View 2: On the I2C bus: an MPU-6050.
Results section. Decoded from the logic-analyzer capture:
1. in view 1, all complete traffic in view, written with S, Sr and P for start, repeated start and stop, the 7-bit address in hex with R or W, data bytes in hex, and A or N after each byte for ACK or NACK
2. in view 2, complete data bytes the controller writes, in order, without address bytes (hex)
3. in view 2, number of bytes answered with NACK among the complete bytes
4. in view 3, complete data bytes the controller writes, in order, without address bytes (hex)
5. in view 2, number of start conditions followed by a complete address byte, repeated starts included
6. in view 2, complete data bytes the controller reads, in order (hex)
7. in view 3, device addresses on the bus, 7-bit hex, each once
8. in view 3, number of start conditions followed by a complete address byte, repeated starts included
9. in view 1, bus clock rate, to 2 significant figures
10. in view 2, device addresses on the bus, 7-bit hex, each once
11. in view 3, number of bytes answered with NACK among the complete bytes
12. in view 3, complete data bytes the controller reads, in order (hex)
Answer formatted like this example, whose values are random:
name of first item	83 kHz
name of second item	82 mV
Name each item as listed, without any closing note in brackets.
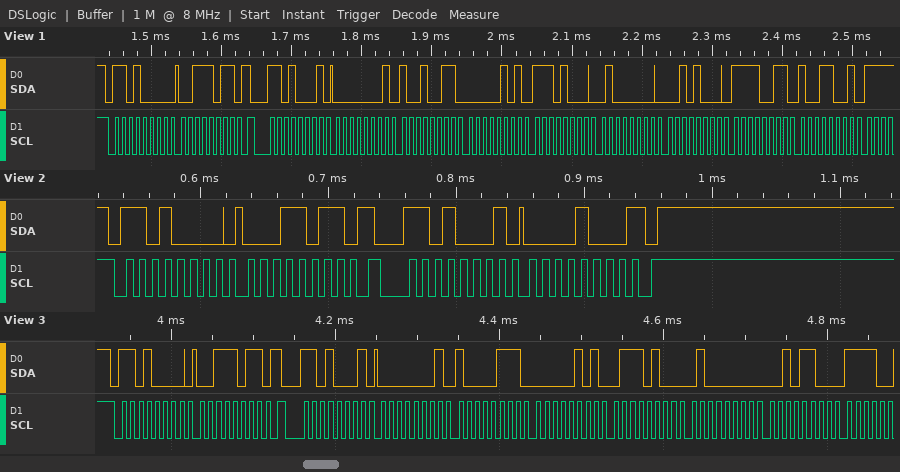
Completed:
in view 1, all complete traffic in view, written with S, Sr and P for start, repeated start and stop, the 7-bit address in hex with R or W, data bytes in hex, and A or N after each byte for ACK or NACK	S 68W A 3B A Sr 68R A 01 A 93 A 05 A E8 A 40 A 28 A F3 A 99 A
in view 2, complete data bytes the controller writes, in order, without address bytes	1B
in view 2, number of bytes answered with NACK among the complete bytes	1
in view 3, complete data bytes the controller writes, in order, without address bytes	3B
in view 2, number of start conditions followed by a complete address byte, repeated starts included	2
in view 2, complete data bytes the controller reads, in order	08
in view 3, device addresses on the bus, 7-bit hex, each once	0x68
in view 3, number of start conditions followed by a complete address byte, repeated starts included	2
in view 1, bus clock rate, to 2 significant figures	100 kHz
in view 2, device addresses on the bus, 7-bit hex, each once	0x68
in view 3, number of bytes answered with NACK among the complete bytes	0
in view 3, complete data bytes the controller reads, in order	01 87 05 74 40 2C
